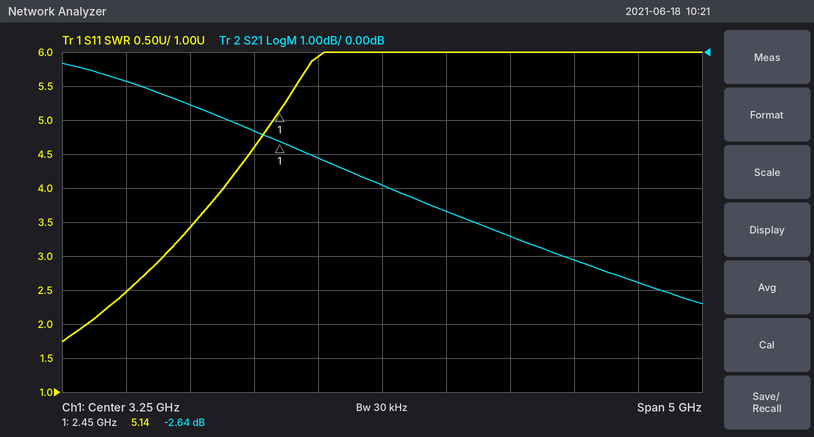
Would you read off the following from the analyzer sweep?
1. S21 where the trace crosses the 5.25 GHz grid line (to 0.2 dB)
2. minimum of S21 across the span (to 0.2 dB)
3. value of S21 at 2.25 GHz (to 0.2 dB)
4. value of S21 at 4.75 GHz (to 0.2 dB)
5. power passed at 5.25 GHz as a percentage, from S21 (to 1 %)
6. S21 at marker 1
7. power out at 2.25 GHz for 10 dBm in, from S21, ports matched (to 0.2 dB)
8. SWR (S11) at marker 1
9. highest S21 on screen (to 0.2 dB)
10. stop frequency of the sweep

-6.8 dB
-7.4 dB
-2.4 dB
-6.2 dB
21 %
-2.64 dB
7.6 dBm
5.14
-0.4 dB
5.75 GHz
